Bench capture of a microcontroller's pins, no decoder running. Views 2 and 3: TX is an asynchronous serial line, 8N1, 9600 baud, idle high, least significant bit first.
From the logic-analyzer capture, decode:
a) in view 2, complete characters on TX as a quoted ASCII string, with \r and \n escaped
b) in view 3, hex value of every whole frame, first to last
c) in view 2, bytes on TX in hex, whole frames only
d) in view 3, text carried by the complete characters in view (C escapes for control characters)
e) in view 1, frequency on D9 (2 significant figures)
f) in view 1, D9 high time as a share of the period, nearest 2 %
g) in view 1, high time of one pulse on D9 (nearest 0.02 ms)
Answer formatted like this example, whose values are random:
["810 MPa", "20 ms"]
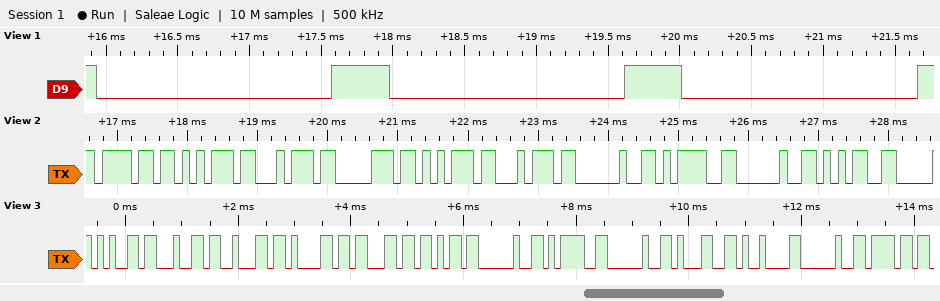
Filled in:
["\"output = 5\"", "65 64 62 61 63 6B 20 3D 20 31 09 20 6F", "0x6F 0x75 0x74 0x70 0x75 0x74 0x20 0x3D 0x20 0x35", "\"edback = 1\\t o\"", "490 Hz", "20 %", "0.40 ms"]
